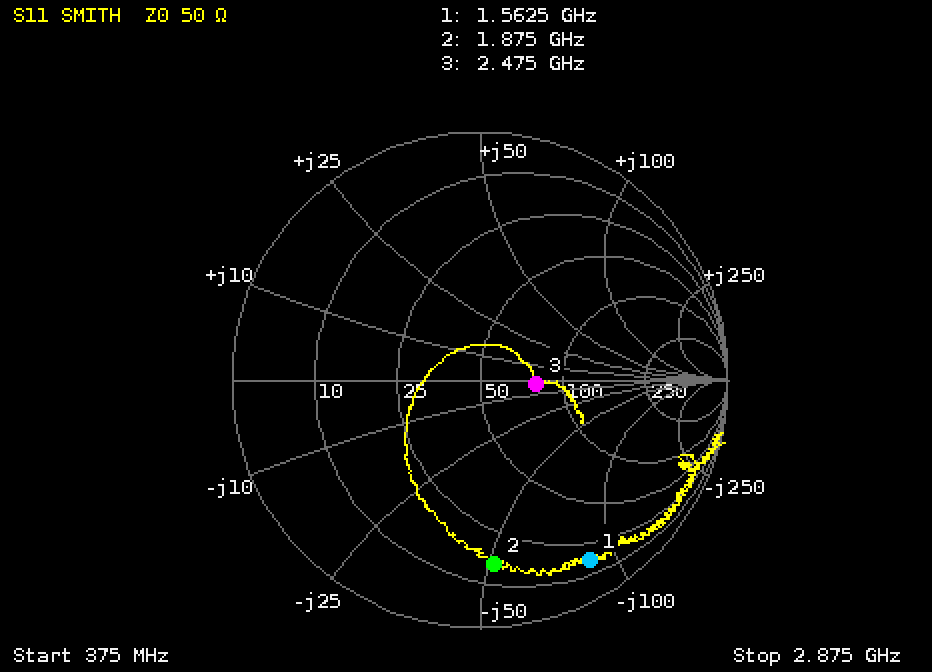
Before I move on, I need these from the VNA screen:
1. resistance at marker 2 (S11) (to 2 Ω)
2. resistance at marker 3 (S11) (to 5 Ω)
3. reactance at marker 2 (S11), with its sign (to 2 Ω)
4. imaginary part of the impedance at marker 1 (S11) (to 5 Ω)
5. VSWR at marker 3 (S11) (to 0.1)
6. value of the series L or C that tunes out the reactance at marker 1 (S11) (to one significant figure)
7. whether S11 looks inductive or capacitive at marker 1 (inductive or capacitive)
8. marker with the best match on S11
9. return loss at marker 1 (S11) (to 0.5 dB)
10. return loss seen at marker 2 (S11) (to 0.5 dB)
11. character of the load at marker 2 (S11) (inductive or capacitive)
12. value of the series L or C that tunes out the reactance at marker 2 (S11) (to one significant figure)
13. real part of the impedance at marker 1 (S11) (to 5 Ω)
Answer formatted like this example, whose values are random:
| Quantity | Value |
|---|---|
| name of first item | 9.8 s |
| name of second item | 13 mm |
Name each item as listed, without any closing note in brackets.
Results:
| Quantity | Value |
|---|---|
| resistance at marker 2 (S11) | 16 Ω |
| resistance at marker 3 (S11) | 80 Ω |
| reactance at marker 2 (S11), with its sign | -52 Ω |
| imaginary part of the impedance at marker 1 (S11) | -85 Ω |
| VSWR at marker 3 (S11) | 1.6 |
| value of the series L or C that tunes out the reactance at marker 1 (S11) | 9 nH |
| whether S11 looks inductive or capacitive at marker 1 | capacitive |
| marker with the best match on S11 | marker 3 |
| return loss at marker 1 (S11) | 1.5 dB |
| return loss seen at marker 2 (S11) | 2.5 dB |
| character of the load at marker 2 (S11) | capacitive |
| value of the series L or C that tunes out the reactance at marker 2 (S11) | 4 nH |
| real part of the impedance at marker 1 (S11) | 15 Ω |
